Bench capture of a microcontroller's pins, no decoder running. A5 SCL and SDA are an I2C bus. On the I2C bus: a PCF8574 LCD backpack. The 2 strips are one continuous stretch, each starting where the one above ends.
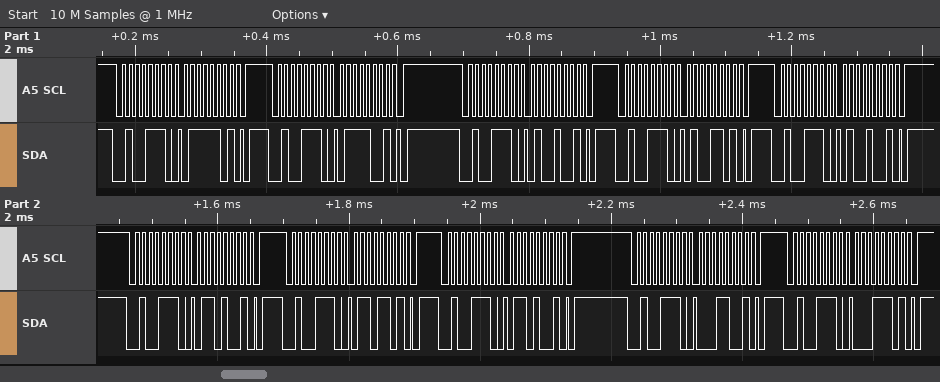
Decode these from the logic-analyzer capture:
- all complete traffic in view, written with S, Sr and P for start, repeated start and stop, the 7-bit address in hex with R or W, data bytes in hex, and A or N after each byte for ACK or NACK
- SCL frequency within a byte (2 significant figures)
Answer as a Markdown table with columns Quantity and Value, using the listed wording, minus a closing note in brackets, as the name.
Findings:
| Quantity | Value |
|---|---|
| all complete traffic in view, written with S, Sr and P for start, repeated start and stop, the 7-bit address in hex with R or W, data bytes in hex, and A or N after each byte for ACK or NACK | S 27W A 7D A P S 27W A 79 A P S 27W A 49 A P S 27W A 4D A P S 27W A 49 A P S 27W A 69 A P S 27W A 6D A P S 27W A 69 A P S 27W A 19 A P S 27W A 1D A P |
| SCL frequency within a byte | 100 kHz |
